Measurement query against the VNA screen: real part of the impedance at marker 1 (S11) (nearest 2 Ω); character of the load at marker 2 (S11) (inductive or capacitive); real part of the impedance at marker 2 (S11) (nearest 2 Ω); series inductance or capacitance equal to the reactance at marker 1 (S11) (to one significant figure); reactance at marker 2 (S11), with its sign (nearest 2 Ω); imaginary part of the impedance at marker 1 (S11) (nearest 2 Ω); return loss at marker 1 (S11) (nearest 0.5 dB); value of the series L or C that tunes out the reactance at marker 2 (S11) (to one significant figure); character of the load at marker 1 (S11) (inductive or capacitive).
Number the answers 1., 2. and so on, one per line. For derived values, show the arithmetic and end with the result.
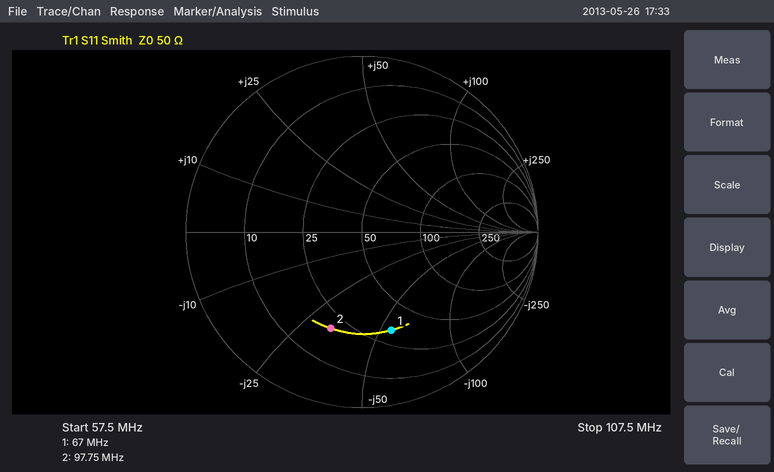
1. 32 Ω
2. capacitive
3. 20 Ω
4. C = 1/(2π × 67 MHz × 56 Ω) ≈ 42.4 pF, so 40 pF to one significant figure
5. -32 Ω
6. -56 Ω
7. 4.5 dB
8. L = 32 Ω/(2π × 97.75 MHz) ≈ 52.1 nH, so 50 nH to one significant figure
9. capacitive
